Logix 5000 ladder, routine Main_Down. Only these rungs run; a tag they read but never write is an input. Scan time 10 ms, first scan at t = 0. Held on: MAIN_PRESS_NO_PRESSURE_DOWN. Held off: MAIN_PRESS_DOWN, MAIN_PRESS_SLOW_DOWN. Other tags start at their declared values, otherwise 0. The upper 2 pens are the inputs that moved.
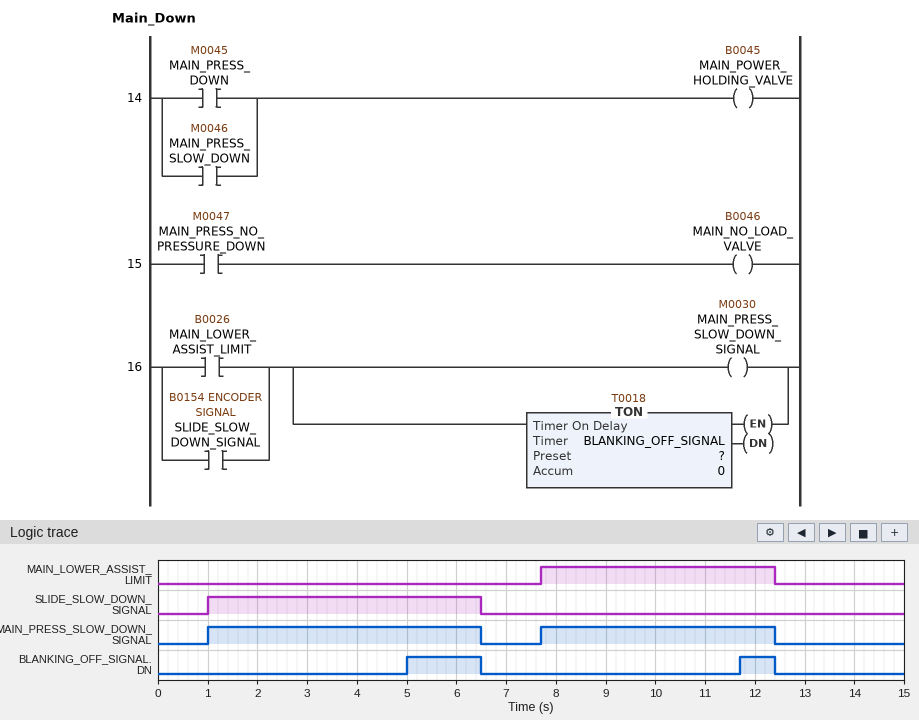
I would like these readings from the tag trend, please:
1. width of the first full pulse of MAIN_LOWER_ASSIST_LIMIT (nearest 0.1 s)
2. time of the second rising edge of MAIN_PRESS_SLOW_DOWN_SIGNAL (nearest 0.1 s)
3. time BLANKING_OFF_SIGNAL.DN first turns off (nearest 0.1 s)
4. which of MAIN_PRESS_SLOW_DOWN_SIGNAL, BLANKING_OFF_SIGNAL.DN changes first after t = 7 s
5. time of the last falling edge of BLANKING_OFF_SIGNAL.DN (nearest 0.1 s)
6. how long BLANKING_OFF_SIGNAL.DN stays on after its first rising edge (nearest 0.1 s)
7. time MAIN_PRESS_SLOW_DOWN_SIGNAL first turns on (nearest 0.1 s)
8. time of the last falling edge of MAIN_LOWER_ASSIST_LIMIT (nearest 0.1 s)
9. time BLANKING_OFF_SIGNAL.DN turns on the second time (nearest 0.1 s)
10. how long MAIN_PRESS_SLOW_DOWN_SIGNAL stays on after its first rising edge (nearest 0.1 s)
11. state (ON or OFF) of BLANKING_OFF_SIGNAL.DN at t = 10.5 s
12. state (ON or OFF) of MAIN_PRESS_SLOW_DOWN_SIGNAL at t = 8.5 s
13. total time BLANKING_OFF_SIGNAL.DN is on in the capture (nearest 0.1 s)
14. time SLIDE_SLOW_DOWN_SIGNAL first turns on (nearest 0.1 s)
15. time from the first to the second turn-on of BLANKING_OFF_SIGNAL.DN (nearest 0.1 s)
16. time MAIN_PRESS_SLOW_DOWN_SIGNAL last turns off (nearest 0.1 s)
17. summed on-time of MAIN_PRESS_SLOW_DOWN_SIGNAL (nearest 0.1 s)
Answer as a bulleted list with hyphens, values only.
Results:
- 4.7 s
- 7.7 s
- 6.5 s
- MAIN_PRESS_SLOW_DOWN_SIGNAL
- 12.4 s
- 1.5 s
- 1.0 s
- 12.4 s
- 11.7 s
- 5.5 s
- OFF
- ON
- 2.2 s
- 1.0 s
- 6.7 s
- 12.4 s
- 10.2 s
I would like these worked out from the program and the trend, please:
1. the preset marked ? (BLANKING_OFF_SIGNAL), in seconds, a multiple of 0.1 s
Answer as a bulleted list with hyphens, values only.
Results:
- 4.0 s
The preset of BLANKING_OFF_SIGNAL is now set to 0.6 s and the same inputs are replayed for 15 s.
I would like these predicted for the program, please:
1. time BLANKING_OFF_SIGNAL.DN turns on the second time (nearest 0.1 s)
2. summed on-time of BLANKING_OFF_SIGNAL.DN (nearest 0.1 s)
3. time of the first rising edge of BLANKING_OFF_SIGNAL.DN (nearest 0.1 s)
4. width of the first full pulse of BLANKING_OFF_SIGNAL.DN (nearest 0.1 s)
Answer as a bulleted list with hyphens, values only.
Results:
- 8.3 s
- 9.0 s
- 1.6 s
- 4.9 s
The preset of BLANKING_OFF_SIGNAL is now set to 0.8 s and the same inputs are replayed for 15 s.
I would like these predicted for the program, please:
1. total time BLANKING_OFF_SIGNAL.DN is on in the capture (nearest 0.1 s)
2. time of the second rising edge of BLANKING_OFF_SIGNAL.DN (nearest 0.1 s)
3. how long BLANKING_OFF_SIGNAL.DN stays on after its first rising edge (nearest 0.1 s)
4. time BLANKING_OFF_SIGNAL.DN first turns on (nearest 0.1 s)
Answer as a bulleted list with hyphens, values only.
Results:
- 8.6 s
- 8.5 s
- 4.7 s
- 1.8 s
